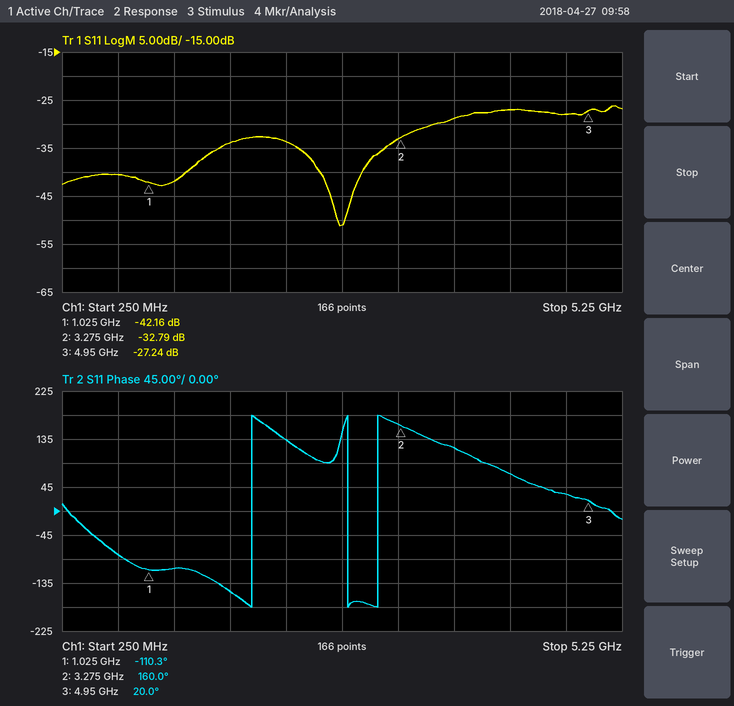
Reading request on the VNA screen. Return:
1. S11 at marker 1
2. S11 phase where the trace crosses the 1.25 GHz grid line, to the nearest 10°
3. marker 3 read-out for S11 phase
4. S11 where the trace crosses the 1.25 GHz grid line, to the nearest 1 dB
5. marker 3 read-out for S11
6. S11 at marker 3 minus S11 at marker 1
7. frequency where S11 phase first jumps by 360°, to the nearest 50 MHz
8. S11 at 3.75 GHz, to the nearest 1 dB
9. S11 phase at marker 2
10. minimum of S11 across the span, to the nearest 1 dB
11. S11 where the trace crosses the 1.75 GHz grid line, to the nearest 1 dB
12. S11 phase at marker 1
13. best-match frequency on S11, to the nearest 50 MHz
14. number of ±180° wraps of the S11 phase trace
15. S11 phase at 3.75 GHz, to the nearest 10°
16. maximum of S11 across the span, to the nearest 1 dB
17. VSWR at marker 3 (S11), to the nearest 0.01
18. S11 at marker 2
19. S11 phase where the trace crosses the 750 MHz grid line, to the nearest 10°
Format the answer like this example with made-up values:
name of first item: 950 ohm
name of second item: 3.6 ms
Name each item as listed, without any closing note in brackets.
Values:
S11 at marker 1: -42.16 dB
S11 phase where the trace crosses the 1.25 GHz grid line, to the nearest 10°: -110°
marker 3 read-out for S11 phase: 20.0°
S11 where the trace crosses the 1.25 GHz grid line, to the nearest 1 dB: -42 dB
marker 3 read-out for S11: -27.24 dB
S11 at marker 3 minus S11 at marker 1: 14.92 dB
frequency where S11 phase first jumps by 360°, to the nearest 50 MHz: 1.95 GHz
S11 at 3.75 GHz, to the nearest 1 dB: -29 dB
S11 phase at marker 2: 160.0°
minimum of S11 across the span, to the nearest 1 dB: -51 dB
S11 where the trace crosses the 1.75 GHz grid line, to the nearest 1 dB: -34 dB
S11 phase at marker 1: -110.3°
best-match frequency on S11, to the nearest 50 MHz: 2.75 GHz
number of ±180° wraps of the S11 phase trace: 3
S11 phase at 3.75 GHz, to the nearest 10°: 120°
maximum of S11 across the span, to the nearest 1 dB: -26 dB
VSWR at marker 3 (S11), to the nearest 0.01: 1.09
S11 at marker 2: -32.79 dB
S11 phase where the trace crosses the 750 MHz grid line, to the nearest 10°: -80°
